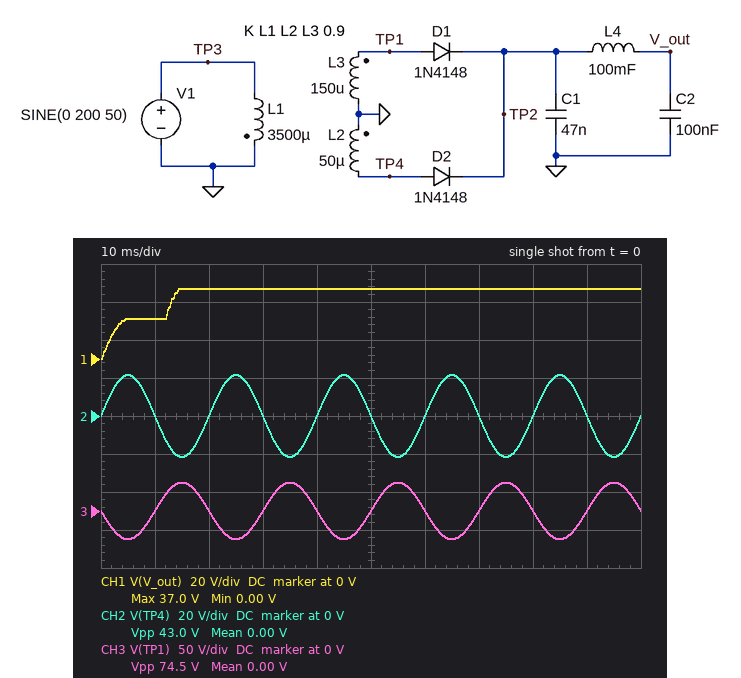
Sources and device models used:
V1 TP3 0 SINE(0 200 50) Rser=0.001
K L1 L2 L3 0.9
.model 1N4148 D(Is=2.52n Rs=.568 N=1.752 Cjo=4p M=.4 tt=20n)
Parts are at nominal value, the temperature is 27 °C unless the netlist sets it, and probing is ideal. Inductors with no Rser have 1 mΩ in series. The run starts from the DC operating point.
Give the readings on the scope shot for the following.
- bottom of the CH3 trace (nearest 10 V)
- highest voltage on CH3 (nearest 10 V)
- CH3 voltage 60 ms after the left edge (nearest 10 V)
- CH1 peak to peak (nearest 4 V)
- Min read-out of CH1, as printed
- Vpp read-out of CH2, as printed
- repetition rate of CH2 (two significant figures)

-40 V
40 V
0 V
36 V
0.00 V
43.0 V
50 Hz
